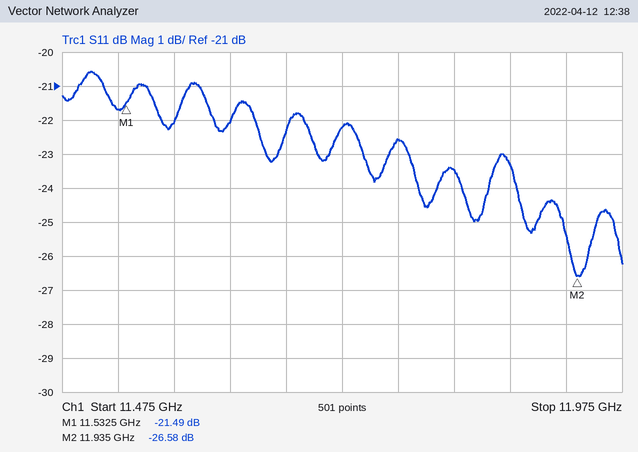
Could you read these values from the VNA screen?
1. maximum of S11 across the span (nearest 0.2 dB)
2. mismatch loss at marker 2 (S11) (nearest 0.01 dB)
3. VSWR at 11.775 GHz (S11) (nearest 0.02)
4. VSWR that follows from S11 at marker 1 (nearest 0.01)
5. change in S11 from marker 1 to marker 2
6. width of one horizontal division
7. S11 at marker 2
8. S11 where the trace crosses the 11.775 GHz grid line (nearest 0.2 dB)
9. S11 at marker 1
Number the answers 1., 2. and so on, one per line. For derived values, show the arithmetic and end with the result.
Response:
1. -20.6 dB
2. −10 log10(1 − 10^(-26.58/10)) ≈ 0.01 dB
3. |Γ| = 10^(-22.6/20) = 0.0741; VSWR = (1 + 0.0741)/(1 − 0.0741) ≈ 1.16
4. (1 + 0.0842)/(1 − 0.0842) ≈ 1.18
5. -26.58 − (-21.49) = -5.09 dB
6. 50 MHz
7. -26.58 dB
8. -22.6 dB
9. -21.49 dB
